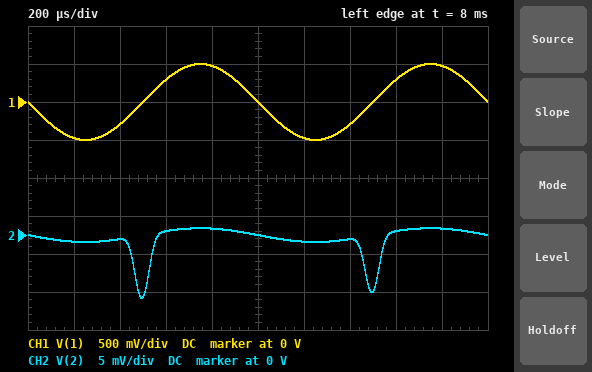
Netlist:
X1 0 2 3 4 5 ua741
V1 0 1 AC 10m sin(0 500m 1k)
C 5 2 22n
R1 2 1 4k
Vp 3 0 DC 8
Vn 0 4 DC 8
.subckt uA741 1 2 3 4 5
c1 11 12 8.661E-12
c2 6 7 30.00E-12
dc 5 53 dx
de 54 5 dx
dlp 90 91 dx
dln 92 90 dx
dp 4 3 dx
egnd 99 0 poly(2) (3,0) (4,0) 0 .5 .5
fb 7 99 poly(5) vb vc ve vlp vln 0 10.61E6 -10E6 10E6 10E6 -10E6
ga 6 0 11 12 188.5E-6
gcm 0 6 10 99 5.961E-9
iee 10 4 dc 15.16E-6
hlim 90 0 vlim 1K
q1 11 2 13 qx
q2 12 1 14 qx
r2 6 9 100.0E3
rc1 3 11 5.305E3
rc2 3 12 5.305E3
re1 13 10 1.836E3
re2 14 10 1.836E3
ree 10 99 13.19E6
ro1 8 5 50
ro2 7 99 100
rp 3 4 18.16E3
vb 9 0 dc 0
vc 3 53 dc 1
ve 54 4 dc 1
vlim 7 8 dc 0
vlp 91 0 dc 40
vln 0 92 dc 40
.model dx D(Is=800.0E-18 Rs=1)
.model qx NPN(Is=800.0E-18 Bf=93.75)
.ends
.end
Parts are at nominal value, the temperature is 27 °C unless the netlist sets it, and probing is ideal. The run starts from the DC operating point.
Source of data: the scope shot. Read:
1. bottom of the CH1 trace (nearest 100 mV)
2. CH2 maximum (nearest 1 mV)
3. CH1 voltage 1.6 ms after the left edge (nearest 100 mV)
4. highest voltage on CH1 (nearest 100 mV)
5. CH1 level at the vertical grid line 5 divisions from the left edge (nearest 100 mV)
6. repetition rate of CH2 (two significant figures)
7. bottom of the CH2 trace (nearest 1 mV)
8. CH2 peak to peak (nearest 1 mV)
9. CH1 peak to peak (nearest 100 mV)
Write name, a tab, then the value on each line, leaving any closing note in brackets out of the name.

bottom of the CH1 trace	-500 mV
CH2 maximum	1 mV
CH1 voltage 1.6 ms after the left edge	300 mV
highest voltage on CH1	500 mV
CH1 level at the vertical grid line 5 divisions from the left edge	0 V
repetition rate of CH2	1.0 kHz
bottom of the CH2 trace	-8 mV
CH2 peak to peak	9 mV
CH1 peak to peak	1.0 V
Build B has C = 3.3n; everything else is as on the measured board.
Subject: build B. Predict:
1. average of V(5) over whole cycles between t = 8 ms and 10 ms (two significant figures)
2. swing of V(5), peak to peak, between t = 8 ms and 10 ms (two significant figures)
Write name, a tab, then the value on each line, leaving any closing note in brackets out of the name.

average of V(5) over whole cycles between t = 8 ms and 10 ms	1.6 V
swing of V(5), peak to peak, between t = 8 ms and 10 ms	12 V
